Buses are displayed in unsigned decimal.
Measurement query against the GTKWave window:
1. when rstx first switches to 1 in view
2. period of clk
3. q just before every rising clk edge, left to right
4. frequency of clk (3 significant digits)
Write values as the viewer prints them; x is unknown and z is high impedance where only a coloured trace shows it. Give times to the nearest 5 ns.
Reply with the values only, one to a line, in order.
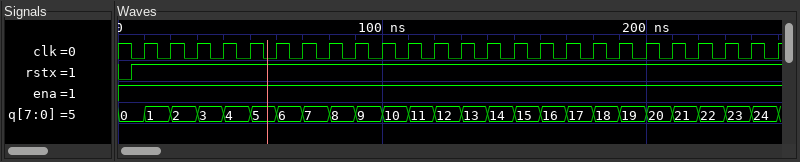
5 ns
10 ns
0, 1, 2, 3, 4, 5, 6, 7, 8, 9, 10, 11, 12, 13, 14, 15, 16, 17, 18, 19, 20, 21, 22, 23, 24
100 MHz
